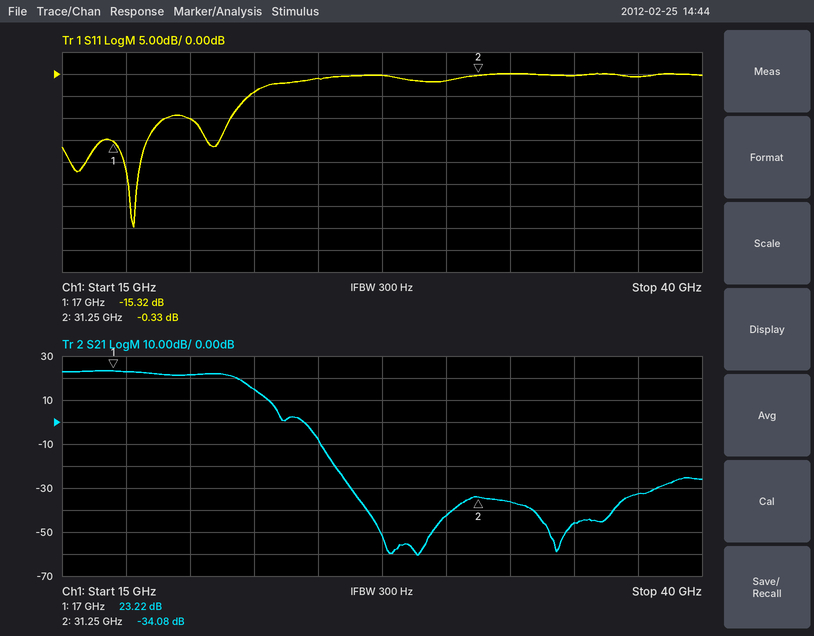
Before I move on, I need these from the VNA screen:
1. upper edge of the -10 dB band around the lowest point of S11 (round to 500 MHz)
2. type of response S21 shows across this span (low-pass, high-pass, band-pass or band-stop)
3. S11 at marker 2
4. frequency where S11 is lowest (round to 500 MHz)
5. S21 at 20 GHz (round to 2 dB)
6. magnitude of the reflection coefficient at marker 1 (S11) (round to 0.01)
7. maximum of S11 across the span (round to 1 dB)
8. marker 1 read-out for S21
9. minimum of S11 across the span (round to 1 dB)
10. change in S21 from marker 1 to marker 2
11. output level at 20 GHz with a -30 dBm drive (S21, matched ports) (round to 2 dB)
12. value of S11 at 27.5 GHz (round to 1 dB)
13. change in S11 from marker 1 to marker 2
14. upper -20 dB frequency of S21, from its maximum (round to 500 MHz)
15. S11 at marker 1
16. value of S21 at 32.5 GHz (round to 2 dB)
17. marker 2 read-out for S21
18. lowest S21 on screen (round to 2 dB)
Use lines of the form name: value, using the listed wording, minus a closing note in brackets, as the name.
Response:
upper edge of the -10 dB band around the lowest point of S11: 19.0 GHz
type of response S21 shows across this span: low-pass
S11 at marker 2: -0.33 dB
frequency where S11 is lowest: 18.0 GHz
S21 at 20 GHz: 22 dB
magnitude of the reflection coefficient at marker 1 (S11): 0.17
maximum of S11 across the span: 0 dB
marker 1 read-out for S21: 23.22 dB
minimum of S11 across the span: -35 dB
change in S21 from marker 1 to marker 2: -57.30 dB
output level at 20 GHz with a -30 dBm drive (S21, matched ports): -8 dBm
value of S11 at 27.5 GHz: 0 dB
change in S11 from marker 1 to marker 2: 14.99 dB
upper -20 dB frequency of S21, from its maximum: 23.5 GHz
S11 at marker 1: -15.32 dB
value of S21 at 32.5 GHz: -36 dB
marker 2 read-out for S21: -34.08 dB
lowest S21 on screen: -60 dB
